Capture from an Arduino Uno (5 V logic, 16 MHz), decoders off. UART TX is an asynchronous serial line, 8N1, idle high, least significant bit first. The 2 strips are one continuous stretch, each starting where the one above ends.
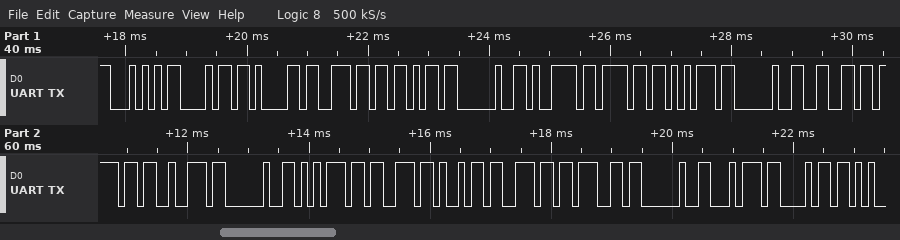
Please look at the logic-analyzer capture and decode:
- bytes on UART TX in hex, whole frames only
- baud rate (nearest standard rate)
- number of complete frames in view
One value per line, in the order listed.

0x54 0x68 0x61 0x6E 0x6B 0x20 0x79 0x6F 0x75 0x20 0x66 0x6F 0x72 0x20 0x75 0x73 0x69 0x6E 0x67 0x20 0x74 0x68
9600 baud
22
